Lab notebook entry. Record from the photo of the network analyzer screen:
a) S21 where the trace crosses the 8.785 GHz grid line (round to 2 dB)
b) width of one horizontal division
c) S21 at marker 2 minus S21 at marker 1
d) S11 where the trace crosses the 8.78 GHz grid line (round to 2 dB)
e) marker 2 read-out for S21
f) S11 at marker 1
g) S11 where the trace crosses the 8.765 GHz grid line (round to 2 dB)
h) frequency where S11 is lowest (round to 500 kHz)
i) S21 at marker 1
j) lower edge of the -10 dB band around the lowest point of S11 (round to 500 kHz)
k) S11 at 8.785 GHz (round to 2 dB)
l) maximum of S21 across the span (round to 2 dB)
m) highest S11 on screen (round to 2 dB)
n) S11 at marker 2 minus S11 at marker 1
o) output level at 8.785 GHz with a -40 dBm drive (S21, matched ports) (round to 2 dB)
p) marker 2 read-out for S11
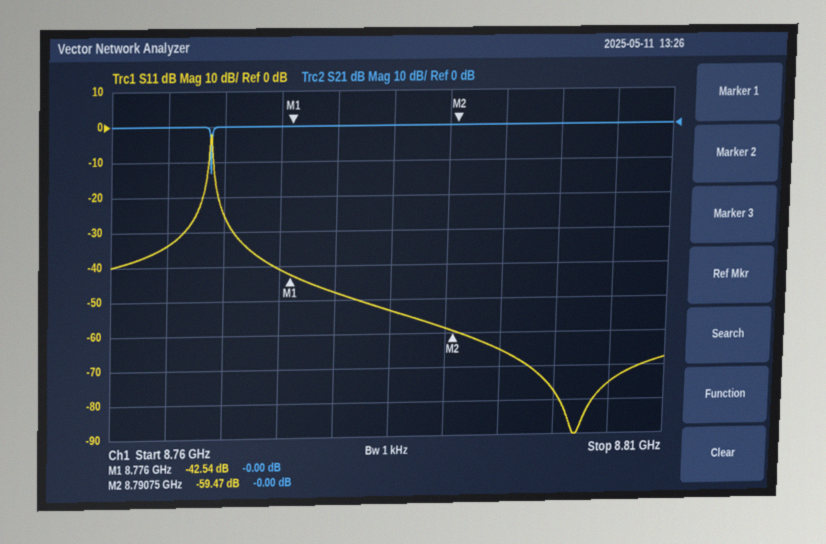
0 dB
5 MHz
0.00 dB
-48 dB
-0.00 dB
-42.54 dB
-34 dB
8.8020 GHz
-0.00 dB
8.7690 GHz
-54 dB
0 dB
-2 dB
-16.93 dB
-40 dBm
-59.47 dB
